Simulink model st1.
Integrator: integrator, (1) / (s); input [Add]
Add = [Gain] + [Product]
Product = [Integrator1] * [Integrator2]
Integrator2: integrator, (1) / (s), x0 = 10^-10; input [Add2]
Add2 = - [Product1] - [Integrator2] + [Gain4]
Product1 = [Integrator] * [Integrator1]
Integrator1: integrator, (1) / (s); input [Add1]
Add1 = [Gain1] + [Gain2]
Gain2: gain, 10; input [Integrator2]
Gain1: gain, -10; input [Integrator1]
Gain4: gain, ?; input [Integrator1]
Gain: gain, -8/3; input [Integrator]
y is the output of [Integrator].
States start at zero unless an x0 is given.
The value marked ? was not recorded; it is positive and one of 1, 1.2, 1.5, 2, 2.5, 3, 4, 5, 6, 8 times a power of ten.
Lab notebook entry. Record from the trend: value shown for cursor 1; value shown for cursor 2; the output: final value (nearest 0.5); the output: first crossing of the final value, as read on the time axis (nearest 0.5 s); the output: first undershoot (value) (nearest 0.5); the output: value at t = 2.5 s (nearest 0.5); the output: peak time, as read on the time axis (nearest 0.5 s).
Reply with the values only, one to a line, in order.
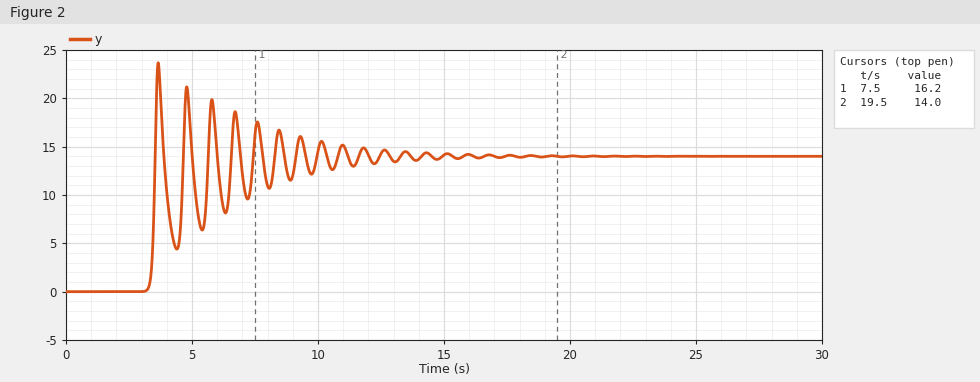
16.2
14.0
14.0
3.5 s
4.5
0.0
3.5 s
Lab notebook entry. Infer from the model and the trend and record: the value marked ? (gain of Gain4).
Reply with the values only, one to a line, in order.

15
